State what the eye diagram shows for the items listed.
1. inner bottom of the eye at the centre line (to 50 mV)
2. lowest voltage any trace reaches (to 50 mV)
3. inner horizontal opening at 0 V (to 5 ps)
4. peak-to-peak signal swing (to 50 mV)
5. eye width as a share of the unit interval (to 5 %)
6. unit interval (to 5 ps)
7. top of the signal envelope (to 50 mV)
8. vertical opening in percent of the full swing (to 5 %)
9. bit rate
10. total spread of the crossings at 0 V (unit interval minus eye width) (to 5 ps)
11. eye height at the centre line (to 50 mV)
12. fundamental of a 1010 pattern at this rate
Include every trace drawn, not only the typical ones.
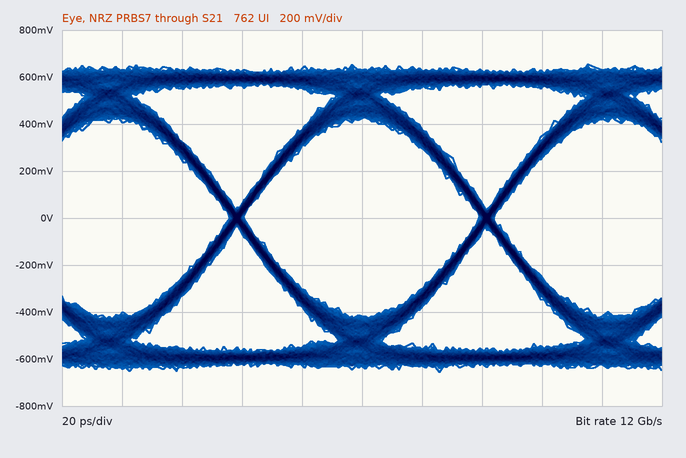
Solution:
-400 mV
-650 mV
80 ps
1.30 V
95 %
85 ps
650 mV
65 %
12 Gb/s
5 ps
850 mV
6 GHz
